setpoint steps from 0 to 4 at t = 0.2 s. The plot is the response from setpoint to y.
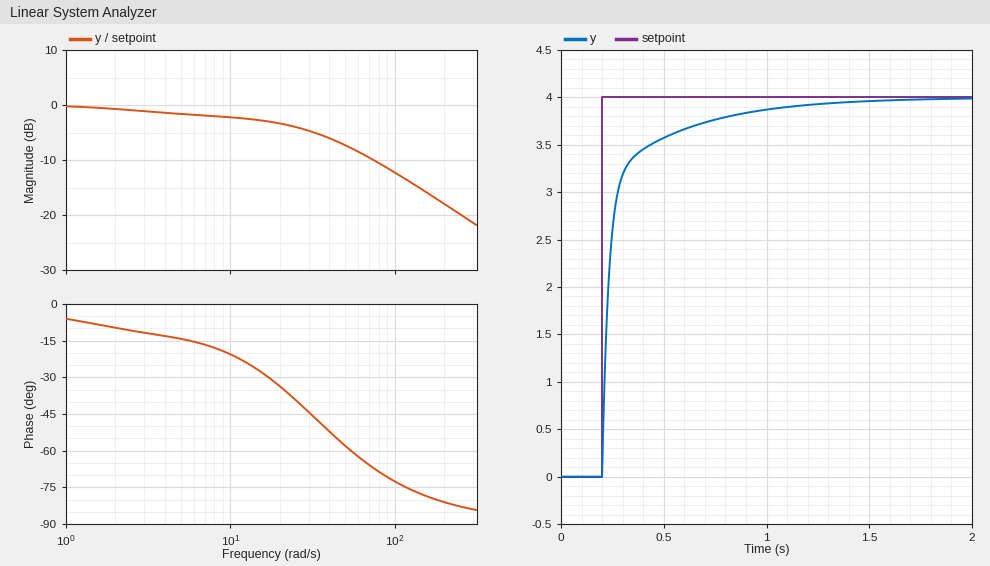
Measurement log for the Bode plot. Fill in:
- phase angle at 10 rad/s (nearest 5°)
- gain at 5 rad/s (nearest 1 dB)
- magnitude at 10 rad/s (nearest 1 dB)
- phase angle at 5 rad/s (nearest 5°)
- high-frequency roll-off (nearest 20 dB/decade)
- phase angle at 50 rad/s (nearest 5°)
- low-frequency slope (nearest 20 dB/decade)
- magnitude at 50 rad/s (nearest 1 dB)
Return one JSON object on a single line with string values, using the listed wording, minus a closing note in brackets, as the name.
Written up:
{"phase angle at 10 rad/s": "-20°", "gain at 5 rad/s": "-2 dB", "magnitude at 10 rad/s": "-2 dB", "phase angle at 5 rad/s": "-15°", "high-frequency roll-off": "-20 dB/decade", "phase angle at 50 rad/s": "-60°", "low-frequency slope": "0 dB/decade", "magnitude at 50 rad/s": "-7 dB"}
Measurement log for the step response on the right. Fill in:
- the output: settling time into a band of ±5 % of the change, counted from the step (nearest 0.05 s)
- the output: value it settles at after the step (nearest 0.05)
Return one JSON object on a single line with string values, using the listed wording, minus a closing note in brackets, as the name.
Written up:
{"the output: settling time into a band of ±5 % of the change, counted from the step": "0.60 s", "the output: value it settles at after the step": "4.00"}
